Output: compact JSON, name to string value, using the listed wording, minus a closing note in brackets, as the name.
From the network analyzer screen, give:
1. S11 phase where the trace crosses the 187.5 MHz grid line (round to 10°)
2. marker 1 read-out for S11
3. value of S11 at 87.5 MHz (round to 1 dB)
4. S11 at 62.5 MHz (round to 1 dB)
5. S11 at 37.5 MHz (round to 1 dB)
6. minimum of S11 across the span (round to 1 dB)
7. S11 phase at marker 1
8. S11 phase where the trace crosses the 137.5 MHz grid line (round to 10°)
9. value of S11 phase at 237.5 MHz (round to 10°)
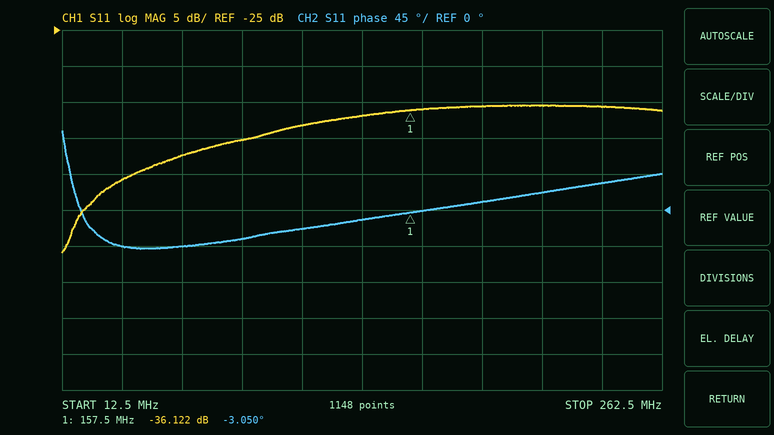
{"S11 phase where the trace crosses the 187.5 MHz grid line": "10°", "marker 1 read-out for S11": "-36.122 dB", "value of S11 at 87.5 MHz": "-40 dB", "S11 at 62.5 MHz": "-42 dB", "S11 at 37.5 MHz": "-46 dB", "minimum of S11 across the span": "-56 dB", "S11 phase at marker 1": "-3.050°", "S11 phase where the trace crosses the 137.5 MHz grid line": "-10°", "value of S11 phase at 237.5 MHz": "30°"}
